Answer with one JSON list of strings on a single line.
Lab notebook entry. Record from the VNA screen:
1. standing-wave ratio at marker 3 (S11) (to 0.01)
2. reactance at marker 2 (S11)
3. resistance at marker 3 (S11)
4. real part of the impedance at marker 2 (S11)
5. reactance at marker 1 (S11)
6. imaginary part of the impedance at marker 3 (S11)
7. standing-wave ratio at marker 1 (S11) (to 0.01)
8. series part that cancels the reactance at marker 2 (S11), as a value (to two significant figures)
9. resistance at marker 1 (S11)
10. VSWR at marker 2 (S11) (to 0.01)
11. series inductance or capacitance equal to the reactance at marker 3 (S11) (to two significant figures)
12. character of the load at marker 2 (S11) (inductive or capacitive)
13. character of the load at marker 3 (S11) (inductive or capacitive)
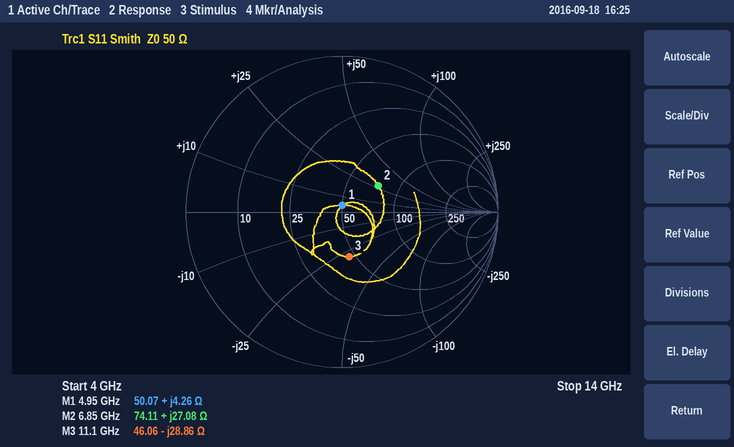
["1.82", "+27.08 Ω", "46.06 Ω", "74.11 Ω", "+4.26 Ω", "-28.86 Ω", "1.09", "860 fF", "50.07 Ω", "1.80", "500 fF", "inductive", "capacitive"]
